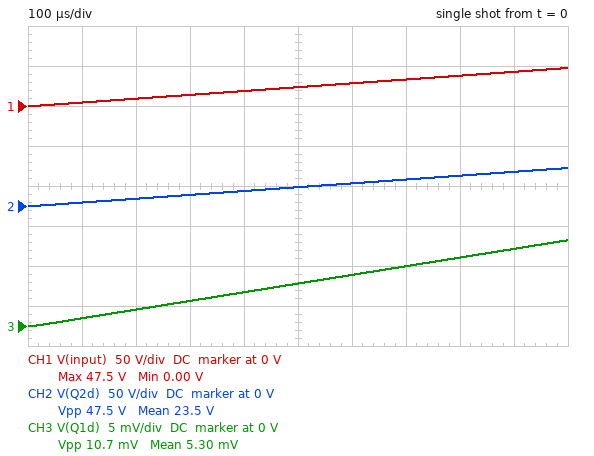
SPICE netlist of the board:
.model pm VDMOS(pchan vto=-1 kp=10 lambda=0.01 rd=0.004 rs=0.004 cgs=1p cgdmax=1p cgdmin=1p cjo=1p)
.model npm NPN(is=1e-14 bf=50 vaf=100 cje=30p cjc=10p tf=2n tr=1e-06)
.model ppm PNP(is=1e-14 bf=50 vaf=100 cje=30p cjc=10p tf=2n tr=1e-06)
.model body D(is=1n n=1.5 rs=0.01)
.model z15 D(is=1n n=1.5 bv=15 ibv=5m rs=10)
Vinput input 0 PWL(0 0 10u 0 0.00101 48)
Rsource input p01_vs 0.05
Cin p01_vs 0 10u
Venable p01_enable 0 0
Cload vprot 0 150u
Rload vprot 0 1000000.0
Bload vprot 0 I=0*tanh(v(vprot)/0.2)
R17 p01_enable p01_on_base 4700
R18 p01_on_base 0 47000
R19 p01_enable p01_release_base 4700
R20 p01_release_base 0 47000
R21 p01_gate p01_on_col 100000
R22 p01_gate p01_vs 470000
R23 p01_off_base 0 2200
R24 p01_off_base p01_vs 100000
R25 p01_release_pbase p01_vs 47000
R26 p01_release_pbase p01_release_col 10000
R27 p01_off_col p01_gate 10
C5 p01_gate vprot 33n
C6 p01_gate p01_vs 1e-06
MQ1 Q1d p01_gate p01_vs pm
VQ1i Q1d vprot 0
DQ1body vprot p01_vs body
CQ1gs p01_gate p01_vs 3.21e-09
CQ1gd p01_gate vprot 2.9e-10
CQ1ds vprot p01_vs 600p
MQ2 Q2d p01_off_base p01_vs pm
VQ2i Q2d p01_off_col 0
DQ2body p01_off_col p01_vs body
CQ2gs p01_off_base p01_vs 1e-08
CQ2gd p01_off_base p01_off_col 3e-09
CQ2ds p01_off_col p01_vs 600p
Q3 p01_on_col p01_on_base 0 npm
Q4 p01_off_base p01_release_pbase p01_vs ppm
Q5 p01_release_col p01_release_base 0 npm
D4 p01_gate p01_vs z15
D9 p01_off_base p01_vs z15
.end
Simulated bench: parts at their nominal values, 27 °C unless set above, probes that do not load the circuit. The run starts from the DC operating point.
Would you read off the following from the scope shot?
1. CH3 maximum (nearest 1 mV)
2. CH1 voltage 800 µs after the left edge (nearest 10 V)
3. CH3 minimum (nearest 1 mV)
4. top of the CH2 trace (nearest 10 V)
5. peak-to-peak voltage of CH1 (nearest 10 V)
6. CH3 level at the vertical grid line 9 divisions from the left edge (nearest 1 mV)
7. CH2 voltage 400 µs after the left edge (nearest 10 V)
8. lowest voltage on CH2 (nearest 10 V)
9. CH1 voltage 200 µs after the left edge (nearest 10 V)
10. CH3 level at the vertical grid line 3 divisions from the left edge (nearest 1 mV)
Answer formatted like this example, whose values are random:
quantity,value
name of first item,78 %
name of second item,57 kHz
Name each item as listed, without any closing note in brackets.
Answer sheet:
quantity,value
CH3 maximum,11 mV
CH1 voltage 800 µs after the left edge,40 V
CH3 minimum,0 V
top of the CH2 trace,50 V
peak-to-peak voltage of CH1,50 V
CH3 level at the vertical grid line 9 divisions from the left edge,10 mV
CH2 voltage 400 µs after the left edge,20 V
lowest voltage on CH2,0 V
CH1 voltage 200 µs after the left edge,10 V
CH3 level at the vertical grid line 3 divisions from the left edge,3 mV
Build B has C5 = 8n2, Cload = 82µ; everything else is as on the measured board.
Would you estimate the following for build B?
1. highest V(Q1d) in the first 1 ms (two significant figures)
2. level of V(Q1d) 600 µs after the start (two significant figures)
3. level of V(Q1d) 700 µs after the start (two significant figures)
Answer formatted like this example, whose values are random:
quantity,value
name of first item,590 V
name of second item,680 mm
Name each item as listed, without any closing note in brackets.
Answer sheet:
quantity,value
highest V(Q1d) in the first 1 ms,5.3 mV
level of V(Q1d) 600 µs after the start,3.1 mV
level of V(Q1d) 700 µs after the start,3.7 mV
